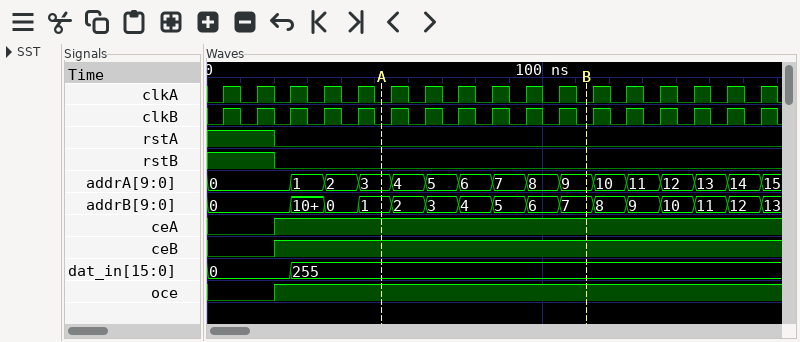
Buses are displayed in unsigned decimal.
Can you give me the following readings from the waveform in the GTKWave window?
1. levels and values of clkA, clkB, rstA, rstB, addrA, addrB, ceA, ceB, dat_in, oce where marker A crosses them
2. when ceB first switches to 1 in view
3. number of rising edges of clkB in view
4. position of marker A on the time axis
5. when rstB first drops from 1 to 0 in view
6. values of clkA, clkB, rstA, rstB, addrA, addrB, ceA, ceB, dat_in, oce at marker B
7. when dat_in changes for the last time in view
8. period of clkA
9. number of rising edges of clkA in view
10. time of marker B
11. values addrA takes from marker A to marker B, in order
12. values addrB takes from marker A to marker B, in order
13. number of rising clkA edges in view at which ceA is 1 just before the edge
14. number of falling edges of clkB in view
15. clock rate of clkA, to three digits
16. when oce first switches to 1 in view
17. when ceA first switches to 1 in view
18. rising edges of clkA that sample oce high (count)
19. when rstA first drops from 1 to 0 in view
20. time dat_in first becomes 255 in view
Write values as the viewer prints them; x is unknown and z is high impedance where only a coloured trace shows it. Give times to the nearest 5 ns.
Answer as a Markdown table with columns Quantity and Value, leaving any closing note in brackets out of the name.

| Quantity | Value |
|---|---|
| levels and values of clkA, clkB, rstA, rstB, addrA, addrB, ceA, ceB, dat_in, oce where marker A crosses them | clkA=0, clkB=0, rstA=0, rstB=0, addrA=3, addrB=1, ceA=1, ceB=1, dat_in=255, oce=1 |
| when ceB first switches to 1 in view | 20 ns |
| number of rising edges of clkB in view | 17 |
| position of marker A on the time axis | 50 ns |
| when rstB first drops from 1 to 0 in view | 20 ns |
| values of clkA, clkB, rstA, rstB, addrA, addrB, ceA, ceB, dat_in, oce at marker B | clkA=0, clkB=0, rstA=0, rstB=0, addrA=9, addrB=7, ceA=1, ceB=1, dat_in=255, oce=1 |
| when dat_in changes for the last time in view | 25 ns |
| period of clkA | 10 ns |
| number of rising edges of clkA in view | 17 |
| time of marker B | 115 ns |
| values addrA takes from marker A to marker B, in order | 3, 4, 5, 6, 7, 8, 9 |
| values addrB takes from marker A to marker B, in order | 1, 2, 3, 4, 5, 6, 7 |
| number of rising clkA edges in view at which ceA is 1 just before the edge | 15 |
| number of falling edges of clkB in view | 17 |
| clock rate of clkA, to three digits | 100 MHz |
| when oce first switches to 1 in view | 20 ns |
| when ceA first switches to 1 in view | 20 ns |
| rising edges of clkA that sample oce high | 15 |
| when rstA first drops from 1 to 0 in view | 20 ns |
| time dat_in first becomes 255 in view | 25 ns |
